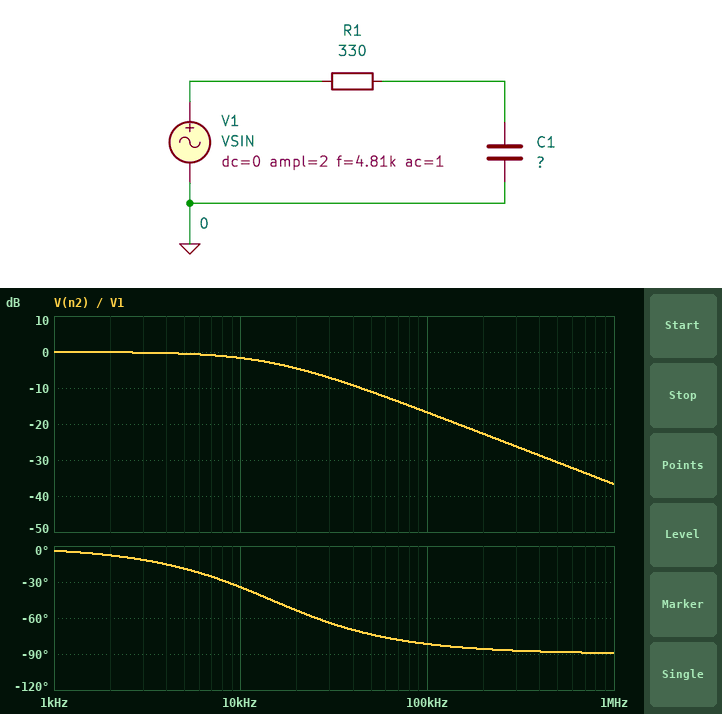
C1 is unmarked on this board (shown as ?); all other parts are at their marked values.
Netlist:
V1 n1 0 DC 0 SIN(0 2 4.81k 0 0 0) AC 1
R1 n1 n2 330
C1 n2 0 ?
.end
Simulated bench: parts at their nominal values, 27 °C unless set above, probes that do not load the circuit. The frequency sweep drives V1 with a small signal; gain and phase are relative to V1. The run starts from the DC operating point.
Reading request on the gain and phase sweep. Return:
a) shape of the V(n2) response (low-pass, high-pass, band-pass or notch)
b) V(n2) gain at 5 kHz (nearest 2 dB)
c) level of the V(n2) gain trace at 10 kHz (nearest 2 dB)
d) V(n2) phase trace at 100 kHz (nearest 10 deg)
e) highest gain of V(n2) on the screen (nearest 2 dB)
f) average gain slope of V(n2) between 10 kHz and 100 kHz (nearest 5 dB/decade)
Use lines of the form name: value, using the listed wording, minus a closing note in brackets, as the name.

shape of the V(n2) response: low-pass
V(n2) gain at 5 kHz: 0 dB
level of the V(n2) gain trace at 10 kHz: -2 dB
V(n2) phase trace at 100 kHz: -80 deg
highest gain of V(n2) on the screen: 0 dB
average gain slope of V(n2) between 10 kHz and 100 kHz: -15 dB/decade
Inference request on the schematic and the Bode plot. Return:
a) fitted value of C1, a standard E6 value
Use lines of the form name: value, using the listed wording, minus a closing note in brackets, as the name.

fitted value of C1, a standard E6 value: 33 nF
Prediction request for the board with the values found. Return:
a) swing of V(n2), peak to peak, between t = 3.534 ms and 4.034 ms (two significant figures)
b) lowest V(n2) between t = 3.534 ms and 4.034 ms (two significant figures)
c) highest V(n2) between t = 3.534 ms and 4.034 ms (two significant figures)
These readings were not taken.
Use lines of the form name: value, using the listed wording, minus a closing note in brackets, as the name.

swing of V(n2), peak to peak, between t = 3.534 ms and 4.034 ms: 3.8 V
lowest V(n2) between t = 3.534 ms and 4.034 ms: -1.9 V
highest V(n2) between t = 3.534 ms and 4.034 ms: 1.9 V
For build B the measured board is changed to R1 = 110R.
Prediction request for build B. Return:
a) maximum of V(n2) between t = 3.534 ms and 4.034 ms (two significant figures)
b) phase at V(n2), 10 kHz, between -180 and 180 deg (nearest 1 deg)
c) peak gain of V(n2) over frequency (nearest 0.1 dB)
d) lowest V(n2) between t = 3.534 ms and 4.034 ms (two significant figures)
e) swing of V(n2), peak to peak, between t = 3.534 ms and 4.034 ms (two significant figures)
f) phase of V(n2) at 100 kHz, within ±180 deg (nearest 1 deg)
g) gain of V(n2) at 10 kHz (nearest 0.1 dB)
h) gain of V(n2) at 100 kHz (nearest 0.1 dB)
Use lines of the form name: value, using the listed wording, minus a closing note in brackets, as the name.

maximum of V(n2) between t = 3.534 ms and 4.034 ms: 2.0 V
phase at V(n2), 10 kHz, between -180 and 180 deg: -13 deg
peak gain of V(n2) over frequency: 0 dB
lowest V(n2) between t = 3.534 ms and 4.034 ms: -2.0 V
swing of V(n2), peak to peak, between t = 3.534 ms and 4.034 ms: 4.0 V
phase of V(n2) at 100 kHz, within ±180 deg: -66 deg
gain of V(n2) at 10 kHz: -0.2 dB
gain of V(n2) at 100 kHz: -7.9 dB
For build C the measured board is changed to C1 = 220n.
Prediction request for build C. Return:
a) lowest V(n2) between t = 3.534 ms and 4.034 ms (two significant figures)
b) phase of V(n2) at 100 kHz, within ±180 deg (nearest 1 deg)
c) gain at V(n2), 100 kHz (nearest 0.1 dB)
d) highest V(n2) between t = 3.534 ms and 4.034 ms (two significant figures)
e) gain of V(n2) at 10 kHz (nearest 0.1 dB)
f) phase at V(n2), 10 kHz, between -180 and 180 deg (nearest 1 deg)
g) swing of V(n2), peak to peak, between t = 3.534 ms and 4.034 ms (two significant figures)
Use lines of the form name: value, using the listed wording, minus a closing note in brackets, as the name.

lowest V(n2) between t = 3.534 ms and 4.034 ms: -830 mV
phase of V(n2) at 100 kHz, within ±180 deg: -89 deg
gain at V(n2), 100 kHz: -33.2 dB
highest V(n2) between t = 3.534 ms and 4.034 ms: 830 mV
gain of V(n2) at 10 kHz: -13.4 dB
phase at V(n2), 10 kHz, between -180 and 180 deg: -78 deg
swing of V(n2), peak to peak, between t = 3.534 ms and 4.034 ms: 1.7 V
